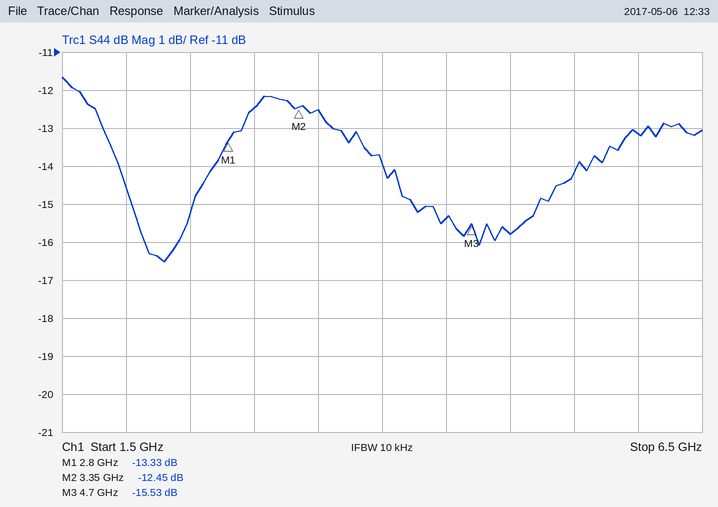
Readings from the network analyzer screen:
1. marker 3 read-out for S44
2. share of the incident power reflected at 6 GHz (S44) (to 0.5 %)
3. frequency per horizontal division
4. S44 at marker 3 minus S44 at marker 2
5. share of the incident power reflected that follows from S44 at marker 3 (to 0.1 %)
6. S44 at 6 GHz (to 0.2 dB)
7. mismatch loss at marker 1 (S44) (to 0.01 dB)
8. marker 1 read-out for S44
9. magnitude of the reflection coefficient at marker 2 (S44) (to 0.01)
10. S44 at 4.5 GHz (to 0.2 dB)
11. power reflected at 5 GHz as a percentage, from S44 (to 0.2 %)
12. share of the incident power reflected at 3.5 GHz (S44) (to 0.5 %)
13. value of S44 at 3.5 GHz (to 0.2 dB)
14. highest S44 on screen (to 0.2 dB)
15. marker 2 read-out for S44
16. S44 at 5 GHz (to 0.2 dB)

-15.53 dB
5.0 %
500 MHz
-3.08 dB
2.8 %
-13.2 dB
0.21 dB
-13.33 dB
0.24
-15.4 dB
2.6 %
5.5 %
-12.6 dB
-11.6 dB
-12.45 dB
-15.8 dB
